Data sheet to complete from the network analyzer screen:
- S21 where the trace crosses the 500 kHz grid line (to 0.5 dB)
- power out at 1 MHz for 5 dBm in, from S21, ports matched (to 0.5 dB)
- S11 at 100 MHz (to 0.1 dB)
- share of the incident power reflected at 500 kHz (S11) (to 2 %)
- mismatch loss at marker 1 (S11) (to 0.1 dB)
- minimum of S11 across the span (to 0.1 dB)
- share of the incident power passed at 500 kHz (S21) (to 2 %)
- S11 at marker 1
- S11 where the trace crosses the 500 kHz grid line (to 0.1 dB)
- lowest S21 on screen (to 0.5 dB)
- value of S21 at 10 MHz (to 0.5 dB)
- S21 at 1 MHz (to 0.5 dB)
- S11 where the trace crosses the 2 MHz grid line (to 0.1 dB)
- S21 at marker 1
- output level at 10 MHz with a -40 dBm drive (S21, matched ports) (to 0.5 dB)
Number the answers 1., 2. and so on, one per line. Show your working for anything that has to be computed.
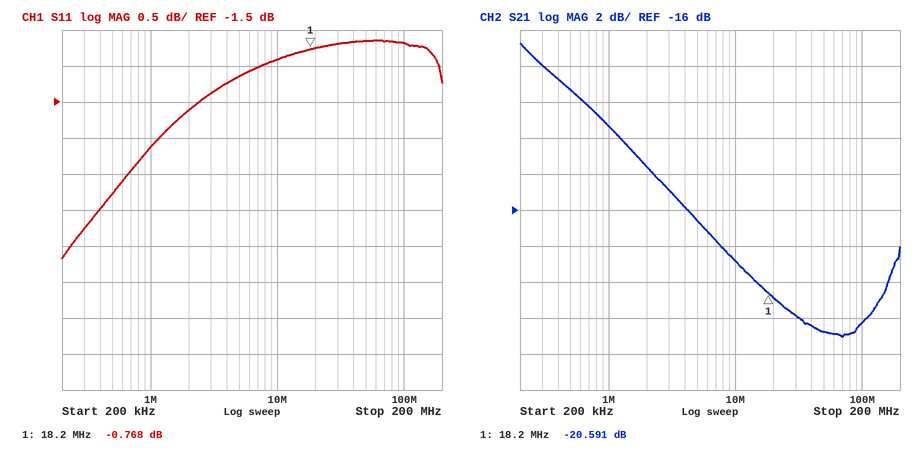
1. -9.5 dB
2. 5 dBm + (-11.5 dB) = -6.5 dBm
3. -0.7 dB
4. 10^(-2.8/10) ≈ 52 %
5. −10 log10(1 − 10^(-0.768/10)) ≈ 7.9 dB
6. -3.7 dB
7. 10^(-9.5/10) ≈ 11.2 %, so 12 % to the nearest 2 %
8. -0.768 dB
9. -2.8 dB
10. -23.0 dB
11. -19.0 dB
12. -11.5 dB
13. -1.6 dB
14. -20.591 dB
15. -40 dBm + (-19.0 dB) = -59.0 dBm
